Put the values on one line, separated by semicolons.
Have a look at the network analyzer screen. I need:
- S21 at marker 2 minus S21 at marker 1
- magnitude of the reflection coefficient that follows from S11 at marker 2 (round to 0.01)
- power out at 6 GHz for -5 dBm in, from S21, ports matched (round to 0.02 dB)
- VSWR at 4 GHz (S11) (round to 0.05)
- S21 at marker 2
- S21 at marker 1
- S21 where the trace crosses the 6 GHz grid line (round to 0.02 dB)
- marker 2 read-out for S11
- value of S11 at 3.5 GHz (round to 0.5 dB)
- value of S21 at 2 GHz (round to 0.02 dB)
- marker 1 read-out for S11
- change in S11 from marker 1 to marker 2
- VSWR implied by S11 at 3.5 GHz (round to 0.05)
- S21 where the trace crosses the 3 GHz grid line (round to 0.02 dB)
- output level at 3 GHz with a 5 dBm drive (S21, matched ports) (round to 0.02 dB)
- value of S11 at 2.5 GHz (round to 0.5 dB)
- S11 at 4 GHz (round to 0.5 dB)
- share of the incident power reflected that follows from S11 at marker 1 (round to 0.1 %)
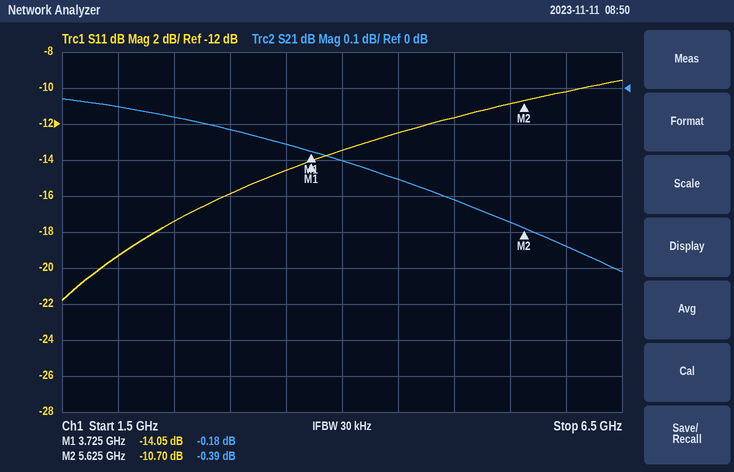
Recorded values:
-0.21 dB; 0.29; -5.44 dBm; 1.55; -0.39 dB; -0.18 dB; -0.44 dB; -10.70 dB; -14.5 dB; -0.06 dB; -14.05 dB; 3.35 dB; 1.45; -0.12 dB; 4.88 dBm; -17.5 dB; -13.5 dB; 3.9 %
